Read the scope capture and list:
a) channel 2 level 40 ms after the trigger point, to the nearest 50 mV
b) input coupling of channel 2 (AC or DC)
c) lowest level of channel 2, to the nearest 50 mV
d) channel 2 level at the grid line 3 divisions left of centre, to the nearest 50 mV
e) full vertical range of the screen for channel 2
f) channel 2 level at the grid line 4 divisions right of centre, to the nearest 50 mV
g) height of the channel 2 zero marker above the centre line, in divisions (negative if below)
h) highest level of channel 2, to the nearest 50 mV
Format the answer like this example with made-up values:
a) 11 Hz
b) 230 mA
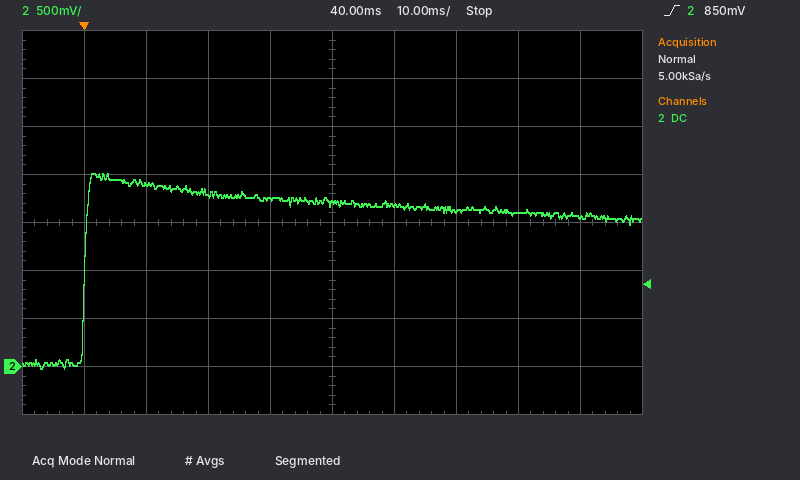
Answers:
a) 1.70 V
b) DC
c) 0 mV
d) 1.90 V
e) 4 V
f) 1.55 V
g) -3.0 div
h) 2.00 V
